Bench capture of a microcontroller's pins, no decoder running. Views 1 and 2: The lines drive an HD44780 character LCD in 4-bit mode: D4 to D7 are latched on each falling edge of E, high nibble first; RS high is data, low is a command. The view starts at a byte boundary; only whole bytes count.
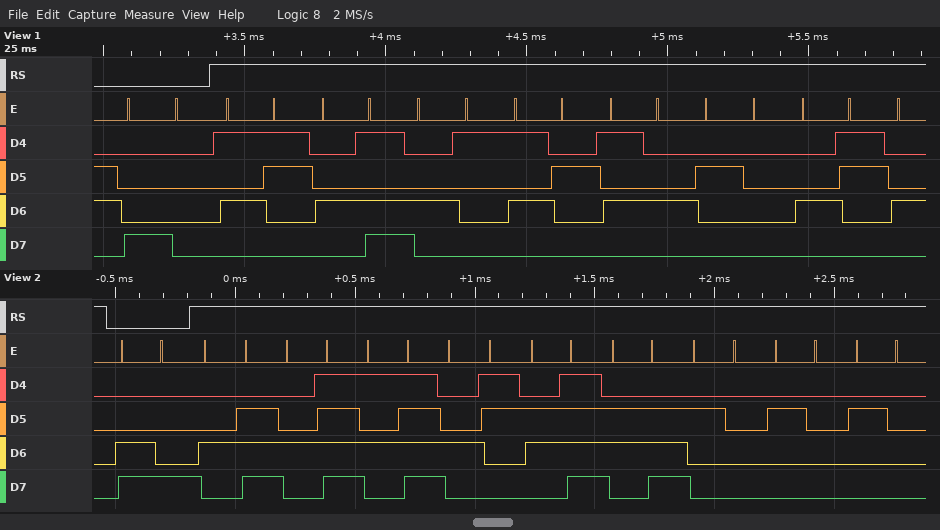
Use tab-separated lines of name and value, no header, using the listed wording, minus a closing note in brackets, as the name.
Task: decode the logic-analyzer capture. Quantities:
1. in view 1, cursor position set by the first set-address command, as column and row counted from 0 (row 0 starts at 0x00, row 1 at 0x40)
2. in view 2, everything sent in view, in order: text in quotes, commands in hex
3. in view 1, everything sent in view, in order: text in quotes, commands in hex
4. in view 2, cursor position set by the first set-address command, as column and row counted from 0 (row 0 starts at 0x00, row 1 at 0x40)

in view 1, cursor position set by the first set-address command, as column and row counted from 0	column 0, row 0
in view 2, everything sent in view, in order: text in quotes, commands in hex	0xC8 "NO_Con   "
in view 1, everything sent in view, in order: text in quotes, commands in hex	0x80 "SMART C"
in view 2, cursor position set by the first set-address command, as column and row counted from 0	column 8, row 1
